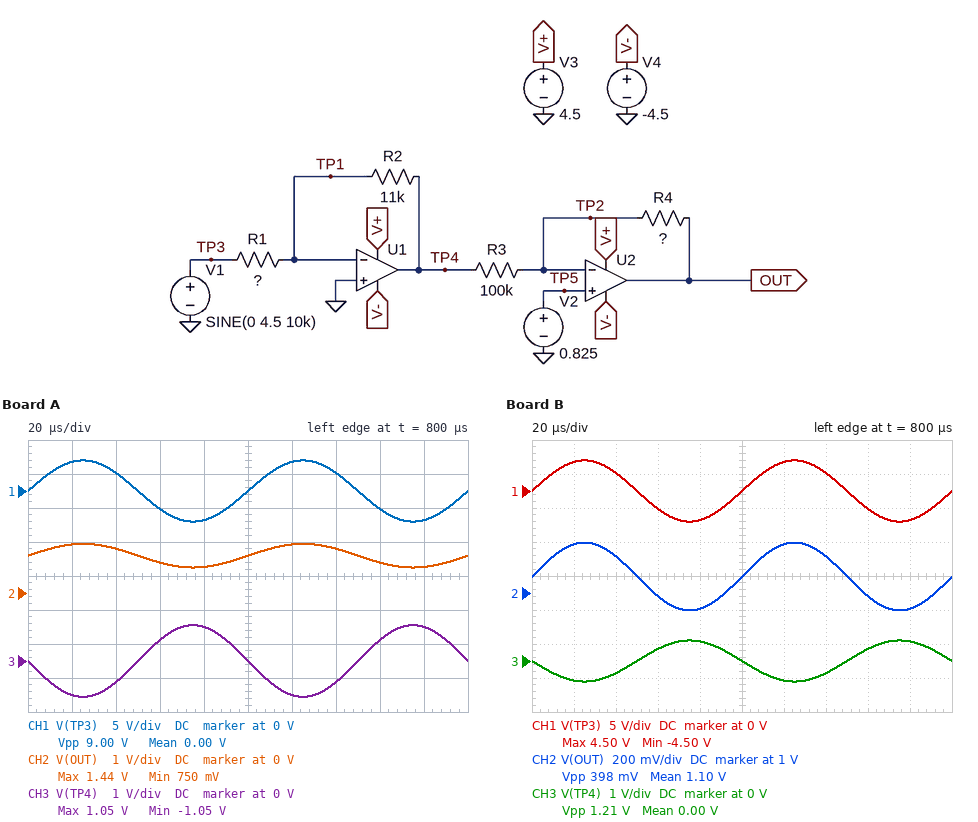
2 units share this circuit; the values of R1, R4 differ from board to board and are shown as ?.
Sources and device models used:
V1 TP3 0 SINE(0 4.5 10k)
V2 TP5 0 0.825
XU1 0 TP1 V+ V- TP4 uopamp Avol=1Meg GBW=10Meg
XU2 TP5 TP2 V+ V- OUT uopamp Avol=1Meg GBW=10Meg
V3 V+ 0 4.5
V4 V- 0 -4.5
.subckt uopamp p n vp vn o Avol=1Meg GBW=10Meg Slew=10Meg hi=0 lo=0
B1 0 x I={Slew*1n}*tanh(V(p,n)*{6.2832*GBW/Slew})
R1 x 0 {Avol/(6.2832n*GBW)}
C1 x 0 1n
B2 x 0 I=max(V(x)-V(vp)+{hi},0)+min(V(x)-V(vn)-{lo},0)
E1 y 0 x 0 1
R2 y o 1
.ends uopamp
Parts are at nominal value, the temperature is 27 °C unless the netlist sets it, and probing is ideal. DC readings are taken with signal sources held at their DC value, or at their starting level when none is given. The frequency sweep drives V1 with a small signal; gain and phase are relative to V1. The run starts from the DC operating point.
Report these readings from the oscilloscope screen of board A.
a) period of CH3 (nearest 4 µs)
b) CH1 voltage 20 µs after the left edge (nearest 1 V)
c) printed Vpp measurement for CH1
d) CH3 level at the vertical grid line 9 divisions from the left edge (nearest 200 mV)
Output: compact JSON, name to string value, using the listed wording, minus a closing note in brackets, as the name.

{"period of CH3": "100 µs", "CH1 voltage 20 µs after the left edge": "4 V", "printed Vpp measurement for CH1": "9.00 V", "CH3 level at the vertical grid line 9 divisions from the left edge": "1.0 V"}
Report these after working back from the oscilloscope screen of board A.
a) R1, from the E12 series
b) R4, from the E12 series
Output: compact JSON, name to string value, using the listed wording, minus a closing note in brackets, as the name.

{"R1, from the E12 series": "47 kΩ", "R4, from the E12 series": "33 kΩ"}
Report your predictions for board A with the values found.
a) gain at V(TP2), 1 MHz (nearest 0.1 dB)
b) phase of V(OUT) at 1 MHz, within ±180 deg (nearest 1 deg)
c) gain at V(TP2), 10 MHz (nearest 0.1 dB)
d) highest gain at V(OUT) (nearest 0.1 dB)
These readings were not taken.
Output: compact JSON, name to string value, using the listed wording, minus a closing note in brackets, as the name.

{"gain at V(TP2), 1 MHz": "-42.4 dB", "phase of V(OUT) at 1 MHz, within ±180 deg": "-15 deg", "gain at V(TP2), 10 MHz": "-30.7 dB", "highest gain at V(OUT)": "-22.2 dB"}
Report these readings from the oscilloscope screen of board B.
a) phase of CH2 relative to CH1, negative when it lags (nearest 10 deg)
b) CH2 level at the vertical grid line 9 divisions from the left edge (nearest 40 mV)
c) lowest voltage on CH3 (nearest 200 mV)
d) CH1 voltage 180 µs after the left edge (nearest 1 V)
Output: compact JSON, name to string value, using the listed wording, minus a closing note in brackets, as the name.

{"phase of CH2 relative to CH1, negative when it lags": "0 deg", "CH2 level at the vertical grid line 9 divisions from the left edge": "920 mV", "lowest voltage on CH3": "-600 mV", "CH1 voltage 180 µs after the left edge": "-4 V"}
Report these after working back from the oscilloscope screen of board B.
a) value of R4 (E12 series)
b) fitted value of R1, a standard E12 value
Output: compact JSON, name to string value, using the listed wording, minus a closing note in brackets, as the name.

{"value of R4": "33 kΩ", "fitted value of R1, a standard E12 value": "82 kΩ"}
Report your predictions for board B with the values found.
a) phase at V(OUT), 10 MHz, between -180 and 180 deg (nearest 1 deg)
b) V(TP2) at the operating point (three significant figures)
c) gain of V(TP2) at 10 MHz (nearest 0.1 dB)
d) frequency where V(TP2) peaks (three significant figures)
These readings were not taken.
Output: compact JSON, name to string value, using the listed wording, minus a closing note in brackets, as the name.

{"phase at V(OUT), 10 MHz, between -180 and 180 deg": "-102 deg", "V(TP2) at the operating point": "825 mV", "gain of V(TP2) at 10 MHz": "-35.1 dB", "frequency where V(TP2) peaks": "8.14 MHz"}
